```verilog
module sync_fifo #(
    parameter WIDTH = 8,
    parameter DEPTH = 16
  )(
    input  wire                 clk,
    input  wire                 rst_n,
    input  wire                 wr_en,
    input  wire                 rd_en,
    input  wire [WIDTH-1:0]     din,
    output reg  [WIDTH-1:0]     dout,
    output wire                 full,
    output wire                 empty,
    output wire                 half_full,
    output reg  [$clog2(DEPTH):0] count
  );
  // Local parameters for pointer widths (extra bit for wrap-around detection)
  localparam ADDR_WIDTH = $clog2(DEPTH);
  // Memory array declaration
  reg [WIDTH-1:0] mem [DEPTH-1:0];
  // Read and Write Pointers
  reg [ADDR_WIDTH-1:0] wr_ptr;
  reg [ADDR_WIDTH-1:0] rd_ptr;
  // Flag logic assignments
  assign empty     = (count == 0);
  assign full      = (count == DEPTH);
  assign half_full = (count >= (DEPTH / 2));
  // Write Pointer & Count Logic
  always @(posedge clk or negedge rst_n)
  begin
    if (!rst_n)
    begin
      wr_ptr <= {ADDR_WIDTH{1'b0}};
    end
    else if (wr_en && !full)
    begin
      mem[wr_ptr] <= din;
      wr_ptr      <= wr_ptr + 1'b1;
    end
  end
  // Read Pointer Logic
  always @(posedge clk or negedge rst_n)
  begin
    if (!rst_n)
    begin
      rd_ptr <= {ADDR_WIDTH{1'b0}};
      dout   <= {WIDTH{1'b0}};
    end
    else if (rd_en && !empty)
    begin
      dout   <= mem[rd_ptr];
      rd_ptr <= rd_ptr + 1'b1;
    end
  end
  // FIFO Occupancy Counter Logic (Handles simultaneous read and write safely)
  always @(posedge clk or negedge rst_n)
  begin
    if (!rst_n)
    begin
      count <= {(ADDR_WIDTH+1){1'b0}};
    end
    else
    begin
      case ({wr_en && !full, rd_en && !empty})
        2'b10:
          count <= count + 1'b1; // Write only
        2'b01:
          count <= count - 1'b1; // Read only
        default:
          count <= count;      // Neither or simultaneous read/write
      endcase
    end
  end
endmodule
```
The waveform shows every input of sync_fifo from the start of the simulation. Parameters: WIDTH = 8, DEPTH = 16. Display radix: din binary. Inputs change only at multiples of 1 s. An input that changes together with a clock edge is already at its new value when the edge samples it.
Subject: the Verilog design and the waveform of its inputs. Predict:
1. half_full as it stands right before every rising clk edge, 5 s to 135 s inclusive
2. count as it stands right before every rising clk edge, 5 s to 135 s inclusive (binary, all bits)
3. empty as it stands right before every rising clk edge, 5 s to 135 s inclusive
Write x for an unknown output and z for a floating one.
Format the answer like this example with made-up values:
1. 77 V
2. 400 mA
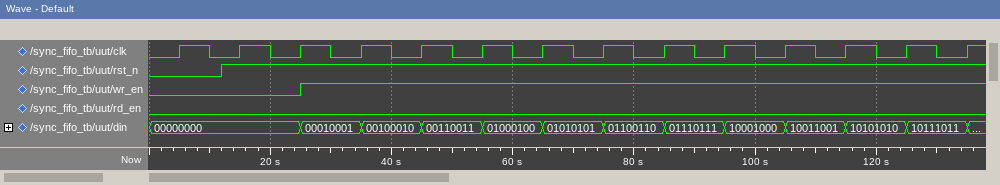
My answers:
1. 0 0 0 0 0 0 0 0 0 0 1 1 1 1
2. 00000, 00000, 00000, 00001, 00010, 00011, 00100, 00101, 00110, 00111, 01000, 01001, 01010, 01011
3. 1 1 1 0 0 0 0 0 0 0 0 0 0 0
